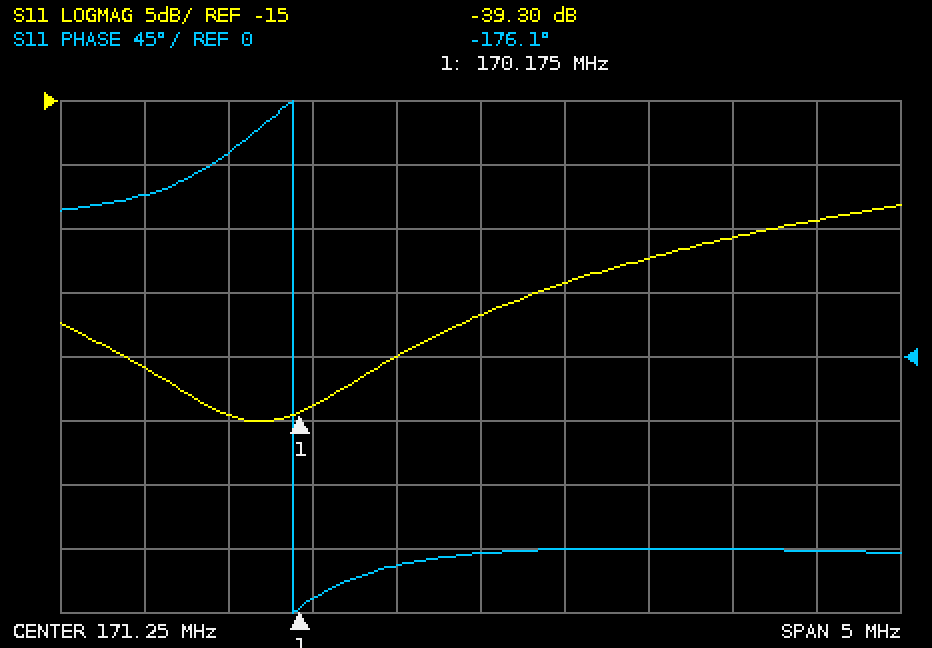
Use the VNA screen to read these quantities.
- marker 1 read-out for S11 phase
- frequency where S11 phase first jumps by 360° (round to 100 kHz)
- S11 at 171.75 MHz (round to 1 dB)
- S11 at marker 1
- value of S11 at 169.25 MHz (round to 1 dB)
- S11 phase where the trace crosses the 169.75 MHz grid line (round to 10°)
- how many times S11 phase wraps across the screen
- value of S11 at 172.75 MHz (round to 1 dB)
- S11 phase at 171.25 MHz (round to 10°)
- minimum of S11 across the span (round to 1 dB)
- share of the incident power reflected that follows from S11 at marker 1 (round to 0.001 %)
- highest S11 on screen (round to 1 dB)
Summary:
-176.1°
170.1 MHz
-29 dB
-39.30 dB
-36 dB
140°
1
-26 dB
-140°
-40 dB
0.012 %
-23 dB
